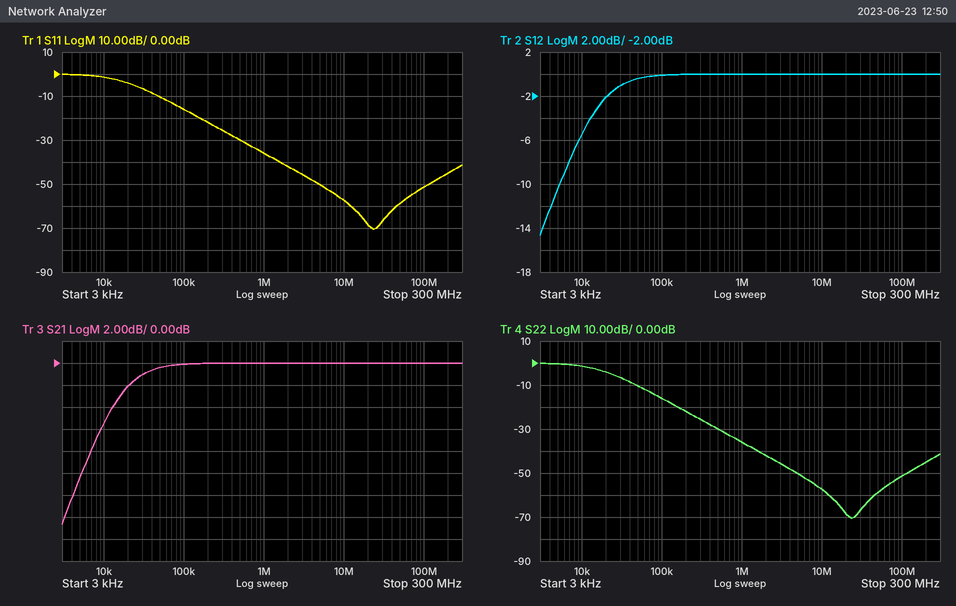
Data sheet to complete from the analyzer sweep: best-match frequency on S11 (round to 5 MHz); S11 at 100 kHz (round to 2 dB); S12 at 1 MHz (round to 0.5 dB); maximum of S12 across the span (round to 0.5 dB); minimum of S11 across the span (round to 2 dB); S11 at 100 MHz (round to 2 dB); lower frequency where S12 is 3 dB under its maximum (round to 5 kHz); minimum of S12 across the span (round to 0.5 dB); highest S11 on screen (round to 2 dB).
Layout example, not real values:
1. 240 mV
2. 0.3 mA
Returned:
1. 25 MHz
2. -16 dB
3. 0.0 dB
4. 0.0 dB
5. -70 dB
6. -52 dB
7. 15 kHz
8. -14.5 dB
9. 0 dB
